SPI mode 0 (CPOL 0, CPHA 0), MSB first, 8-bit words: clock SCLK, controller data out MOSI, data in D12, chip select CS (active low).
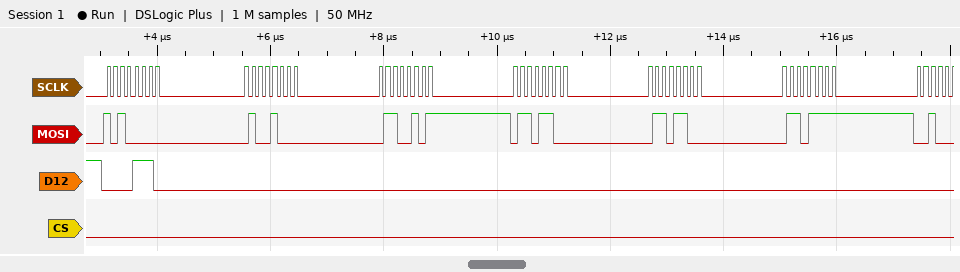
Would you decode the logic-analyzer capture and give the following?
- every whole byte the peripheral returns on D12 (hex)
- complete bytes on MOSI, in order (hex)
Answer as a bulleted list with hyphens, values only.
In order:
- 0E 00 00 00 00 00
- A0 48 65 6C 6C 6F
